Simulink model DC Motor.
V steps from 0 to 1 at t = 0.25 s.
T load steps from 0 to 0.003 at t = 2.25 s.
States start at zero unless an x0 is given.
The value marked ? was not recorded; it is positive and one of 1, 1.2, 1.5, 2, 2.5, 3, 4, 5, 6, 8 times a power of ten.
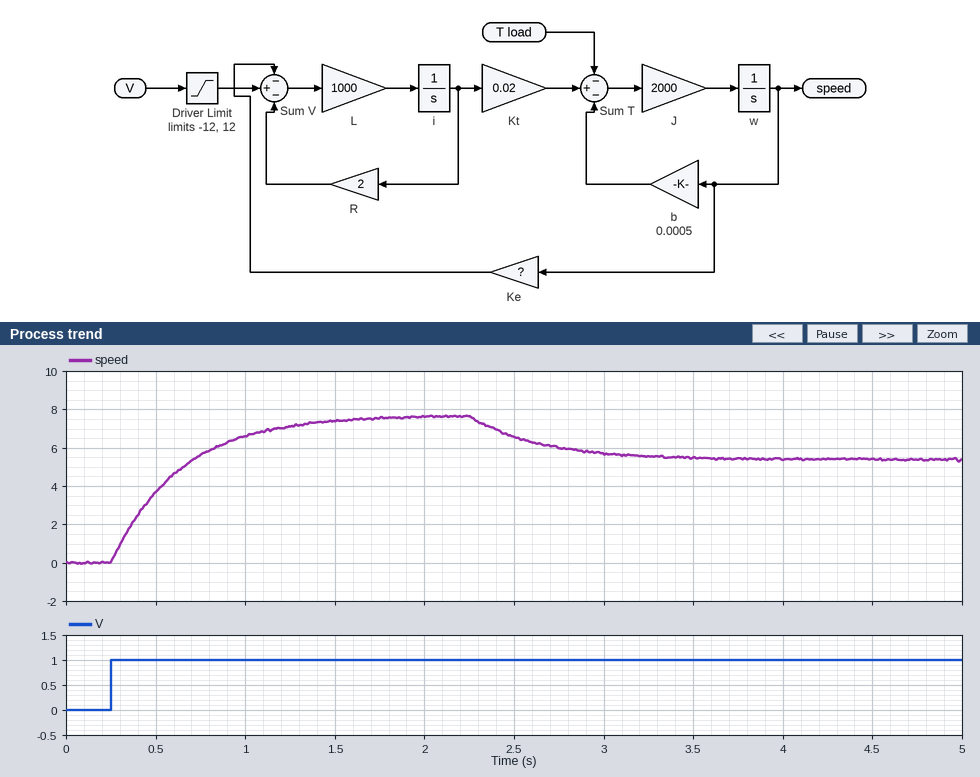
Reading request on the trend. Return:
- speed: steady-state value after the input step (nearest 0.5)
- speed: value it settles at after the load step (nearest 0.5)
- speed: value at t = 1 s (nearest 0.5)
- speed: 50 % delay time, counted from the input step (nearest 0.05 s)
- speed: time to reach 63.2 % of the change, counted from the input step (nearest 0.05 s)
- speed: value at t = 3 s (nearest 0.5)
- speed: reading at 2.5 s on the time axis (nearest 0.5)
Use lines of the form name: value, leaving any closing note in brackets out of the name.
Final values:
speed: steady-state value after the input step: 7.5
speed: value it settles at after the load step: 5.5
speed: value at t = 1 s: 6.5
speed: 50 % delay time, counted from the input step: 0.25 s
speed: time to reach 63.2 % of the change, counted from the input step: 0.40 s
speed: value at t = 3 s: 5.5
speed: reading at 2.5 s on the time axis: 6.5
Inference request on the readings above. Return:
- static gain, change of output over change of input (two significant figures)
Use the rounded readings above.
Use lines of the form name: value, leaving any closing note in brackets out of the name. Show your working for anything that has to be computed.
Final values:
static gain, change of output over change of input: (7.5 - 0) / (1 - 0) = 7.5
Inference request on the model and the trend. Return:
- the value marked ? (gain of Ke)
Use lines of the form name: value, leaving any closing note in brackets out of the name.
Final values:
the value marked ?: 0.08
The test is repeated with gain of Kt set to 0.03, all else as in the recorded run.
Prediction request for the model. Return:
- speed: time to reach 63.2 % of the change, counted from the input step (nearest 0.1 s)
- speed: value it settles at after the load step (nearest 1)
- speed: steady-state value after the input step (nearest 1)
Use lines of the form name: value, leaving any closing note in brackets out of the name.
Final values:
speed: time to reach 63.2 % of the change, counted from the input step: 0.3 s
speed: value it settles at after the load step: 7
speed: steady-state value after the input step: 9
